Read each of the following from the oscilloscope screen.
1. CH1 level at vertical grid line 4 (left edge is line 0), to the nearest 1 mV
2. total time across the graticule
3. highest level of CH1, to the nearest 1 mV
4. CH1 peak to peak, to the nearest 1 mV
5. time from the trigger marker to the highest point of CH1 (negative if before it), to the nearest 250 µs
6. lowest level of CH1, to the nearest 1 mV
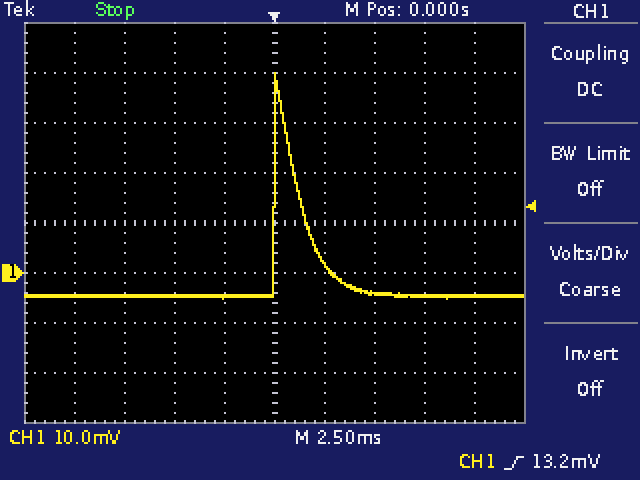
-5 mV
25 ms
40 mV
45 mV
0.00 ms
-5 mV
